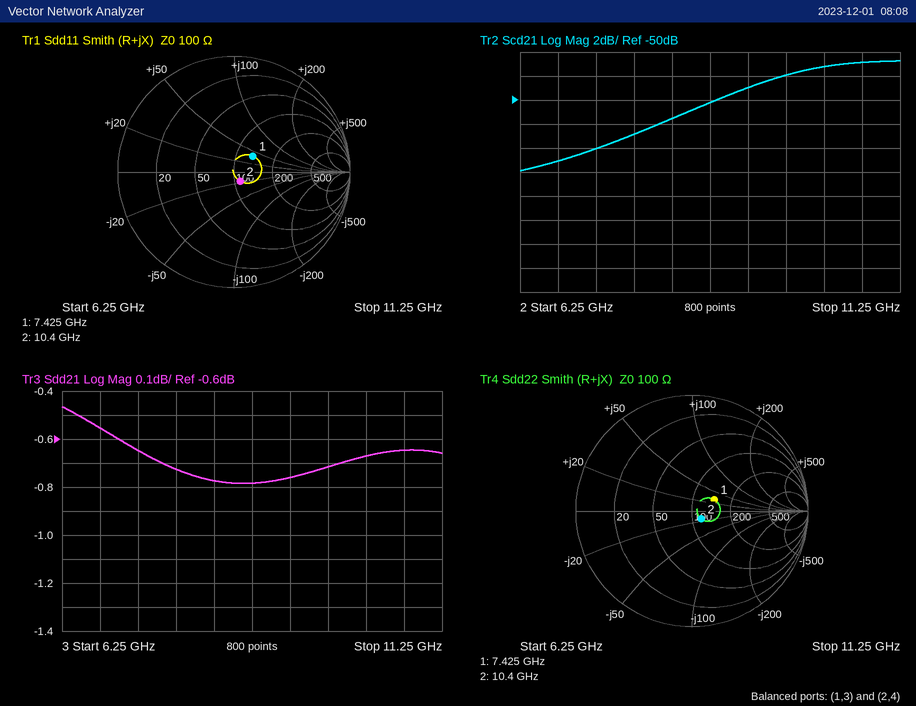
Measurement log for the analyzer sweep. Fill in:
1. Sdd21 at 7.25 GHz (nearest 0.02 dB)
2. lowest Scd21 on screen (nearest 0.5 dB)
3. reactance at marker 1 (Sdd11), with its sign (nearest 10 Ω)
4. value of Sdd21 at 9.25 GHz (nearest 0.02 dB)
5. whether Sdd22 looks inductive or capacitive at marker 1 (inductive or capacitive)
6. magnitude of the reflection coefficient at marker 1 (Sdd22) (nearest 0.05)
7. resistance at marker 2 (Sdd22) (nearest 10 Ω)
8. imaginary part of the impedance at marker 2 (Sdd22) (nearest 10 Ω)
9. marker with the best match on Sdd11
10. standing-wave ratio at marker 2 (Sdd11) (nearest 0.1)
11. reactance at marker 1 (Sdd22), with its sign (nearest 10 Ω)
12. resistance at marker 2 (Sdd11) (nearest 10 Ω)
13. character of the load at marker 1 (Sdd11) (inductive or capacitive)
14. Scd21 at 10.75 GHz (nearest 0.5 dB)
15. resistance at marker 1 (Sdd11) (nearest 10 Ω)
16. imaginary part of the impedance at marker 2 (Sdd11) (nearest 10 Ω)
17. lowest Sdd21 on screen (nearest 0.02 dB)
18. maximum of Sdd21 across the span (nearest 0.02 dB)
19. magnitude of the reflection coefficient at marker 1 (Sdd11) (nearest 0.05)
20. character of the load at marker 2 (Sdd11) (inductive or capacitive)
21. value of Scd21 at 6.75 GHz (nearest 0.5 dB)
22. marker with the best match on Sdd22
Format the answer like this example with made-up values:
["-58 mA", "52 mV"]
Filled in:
["-0.64 dB", "-56.0 dB", "+40 Ω", "-0.76 dB", "inductive", "0.20", "120 Ω", "-20 Ω", "marker 2", "1.2", "+30 Ω", "110 Ω", "inductive", "-47.0 dB", "130 Ω", "-20 Ω", "-0.78 dB", "-0.46 dB", "0.20", "capacitive", "-55.0 dB", "marker 2"]
